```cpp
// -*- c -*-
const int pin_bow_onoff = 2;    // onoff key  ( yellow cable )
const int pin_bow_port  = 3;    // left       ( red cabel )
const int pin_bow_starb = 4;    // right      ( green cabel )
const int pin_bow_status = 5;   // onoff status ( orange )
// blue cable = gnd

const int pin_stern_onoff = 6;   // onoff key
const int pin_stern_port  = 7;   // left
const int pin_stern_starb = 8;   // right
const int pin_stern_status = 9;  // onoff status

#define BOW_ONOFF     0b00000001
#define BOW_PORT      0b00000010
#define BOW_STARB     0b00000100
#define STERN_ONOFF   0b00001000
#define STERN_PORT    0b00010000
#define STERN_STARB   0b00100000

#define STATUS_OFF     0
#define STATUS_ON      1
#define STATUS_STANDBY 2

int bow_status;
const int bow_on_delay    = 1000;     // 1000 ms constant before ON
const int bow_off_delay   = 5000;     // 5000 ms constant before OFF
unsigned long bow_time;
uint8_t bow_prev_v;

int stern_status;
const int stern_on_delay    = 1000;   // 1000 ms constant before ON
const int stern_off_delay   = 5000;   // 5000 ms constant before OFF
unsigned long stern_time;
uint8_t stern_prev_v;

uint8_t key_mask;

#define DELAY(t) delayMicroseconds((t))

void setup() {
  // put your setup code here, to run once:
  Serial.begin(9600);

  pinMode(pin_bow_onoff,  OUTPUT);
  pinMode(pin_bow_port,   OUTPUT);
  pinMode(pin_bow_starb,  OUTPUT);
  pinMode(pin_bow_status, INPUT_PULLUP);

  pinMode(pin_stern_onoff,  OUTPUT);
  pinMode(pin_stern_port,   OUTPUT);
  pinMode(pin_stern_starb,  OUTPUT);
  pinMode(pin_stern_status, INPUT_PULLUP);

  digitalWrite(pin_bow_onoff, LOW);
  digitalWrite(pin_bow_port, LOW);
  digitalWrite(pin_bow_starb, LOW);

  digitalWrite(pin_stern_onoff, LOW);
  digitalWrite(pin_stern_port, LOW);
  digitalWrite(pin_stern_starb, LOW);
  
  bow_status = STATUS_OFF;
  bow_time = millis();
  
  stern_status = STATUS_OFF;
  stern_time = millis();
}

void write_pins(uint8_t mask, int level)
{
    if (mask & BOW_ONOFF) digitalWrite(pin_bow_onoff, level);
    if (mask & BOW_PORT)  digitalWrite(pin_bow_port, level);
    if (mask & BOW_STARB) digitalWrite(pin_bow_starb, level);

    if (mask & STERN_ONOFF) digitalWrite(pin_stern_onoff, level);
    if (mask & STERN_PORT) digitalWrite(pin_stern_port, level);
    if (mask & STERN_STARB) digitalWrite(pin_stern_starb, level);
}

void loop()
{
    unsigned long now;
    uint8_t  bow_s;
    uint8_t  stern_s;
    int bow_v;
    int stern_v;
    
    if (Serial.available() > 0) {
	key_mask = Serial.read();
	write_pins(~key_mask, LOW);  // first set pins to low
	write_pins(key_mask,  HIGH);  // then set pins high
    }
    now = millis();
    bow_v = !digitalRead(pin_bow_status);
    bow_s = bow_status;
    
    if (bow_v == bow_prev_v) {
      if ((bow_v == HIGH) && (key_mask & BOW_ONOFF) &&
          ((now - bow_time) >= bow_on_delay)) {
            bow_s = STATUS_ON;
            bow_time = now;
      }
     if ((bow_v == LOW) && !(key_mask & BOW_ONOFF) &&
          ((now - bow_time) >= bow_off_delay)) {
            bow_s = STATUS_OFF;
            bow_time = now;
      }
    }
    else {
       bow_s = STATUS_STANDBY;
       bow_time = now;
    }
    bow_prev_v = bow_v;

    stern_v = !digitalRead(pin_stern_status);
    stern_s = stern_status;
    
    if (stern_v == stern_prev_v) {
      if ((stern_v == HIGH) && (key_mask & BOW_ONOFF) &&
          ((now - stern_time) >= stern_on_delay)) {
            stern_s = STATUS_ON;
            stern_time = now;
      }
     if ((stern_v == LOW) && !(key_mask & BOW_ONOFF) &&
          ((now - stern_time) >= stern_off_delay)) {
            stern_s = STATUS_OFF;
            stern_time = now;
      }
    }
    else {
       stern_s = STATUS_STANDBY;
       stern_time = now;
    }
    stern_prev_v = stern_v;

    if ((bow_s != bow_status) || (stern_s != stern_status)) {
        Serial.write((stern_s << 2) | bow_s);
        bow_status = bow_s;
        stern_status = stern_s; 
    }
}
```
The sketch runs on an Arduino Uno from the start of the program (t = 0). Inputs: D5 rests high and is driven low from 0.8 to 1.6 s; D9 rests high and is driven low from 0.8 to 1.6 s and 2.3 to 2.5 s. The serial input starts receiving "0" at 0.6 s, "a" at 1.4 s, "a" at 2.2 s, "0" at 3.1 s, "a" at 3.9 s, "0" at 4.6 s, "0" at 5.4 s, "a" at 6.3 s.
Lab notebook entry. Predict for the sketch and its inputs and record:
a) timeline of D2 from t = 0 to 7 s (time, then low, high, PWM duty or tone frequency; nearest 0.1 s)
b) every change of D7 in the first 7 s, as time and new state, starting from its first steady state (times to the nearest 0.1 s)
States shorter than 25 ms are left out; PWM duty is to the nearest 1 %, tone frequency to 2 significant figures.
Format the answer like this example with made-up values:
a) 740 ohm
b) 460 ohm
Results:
a) 0 s low; 1.4 s high; 3.1 s low; 3.9 s high; 4.6 s low; 6.3 s high
b) 0 s low; 0.6 s high; 1.4 s low; 3.1 s high; 3.9 s low; 4.6 s high; 6.3 s low
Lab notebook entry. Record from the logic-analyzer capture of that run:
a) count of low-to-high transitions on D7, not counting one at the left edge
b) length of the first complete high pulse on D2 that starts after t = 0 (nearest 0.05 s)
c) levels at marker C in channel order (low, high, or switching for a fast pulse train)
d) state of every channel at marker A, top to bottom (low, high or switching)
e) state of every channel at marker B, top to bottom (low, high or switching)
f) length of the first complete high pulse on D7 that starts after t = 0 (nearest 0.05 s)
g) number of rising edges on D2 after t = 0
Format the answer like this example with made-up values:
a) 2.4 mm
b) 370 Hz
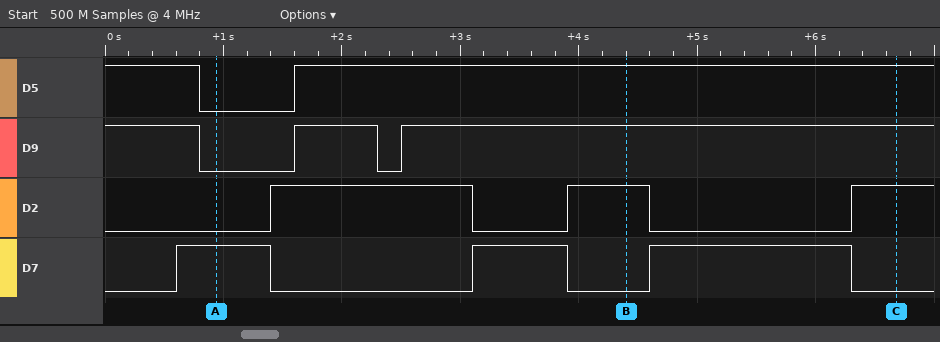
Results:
a) 3
b) 1.70 s
c) D5 high, D9 high, D2 high, D7 low
d) D5 low, D9 low, D2 low, D7 high
e) D5 high, D9 high, D2 high, D7 low
f) 0.80 s
g) 3
